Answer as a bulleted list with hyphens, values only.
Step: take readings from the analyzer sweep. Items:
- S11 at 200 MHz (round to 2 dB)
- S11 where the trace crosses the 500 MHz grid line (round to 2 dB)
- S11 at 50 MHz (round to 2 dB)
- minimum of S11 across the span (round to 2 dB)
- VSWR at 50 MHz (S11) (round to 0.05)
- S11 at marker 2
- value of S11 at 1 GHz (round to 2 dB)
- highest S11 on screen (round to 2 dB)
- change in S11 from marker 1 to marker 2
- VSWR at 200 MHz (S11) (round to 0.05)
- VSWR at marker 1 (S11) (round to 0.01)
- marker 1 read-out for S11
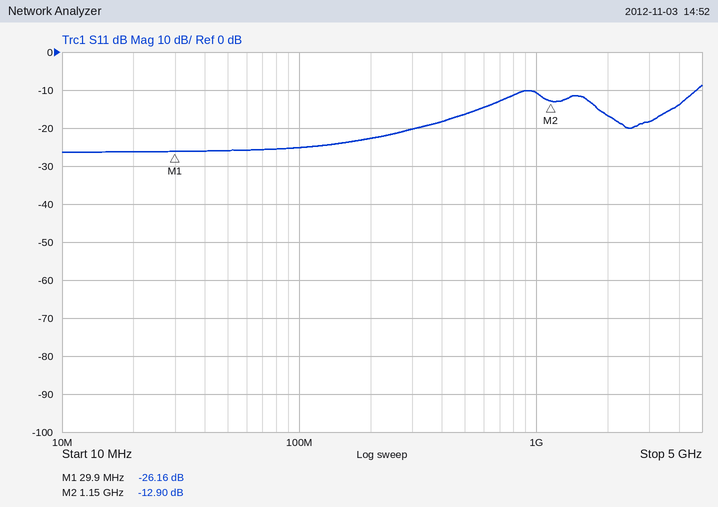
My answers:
- -22 dB
- -16 dB
- -26 dB
- -26 dB
- 1.10
- -12.90 dB
- -10 dB
- -8 dB
- 13.26 dB
- 1.15
- 1.10
- -26.16 dB
